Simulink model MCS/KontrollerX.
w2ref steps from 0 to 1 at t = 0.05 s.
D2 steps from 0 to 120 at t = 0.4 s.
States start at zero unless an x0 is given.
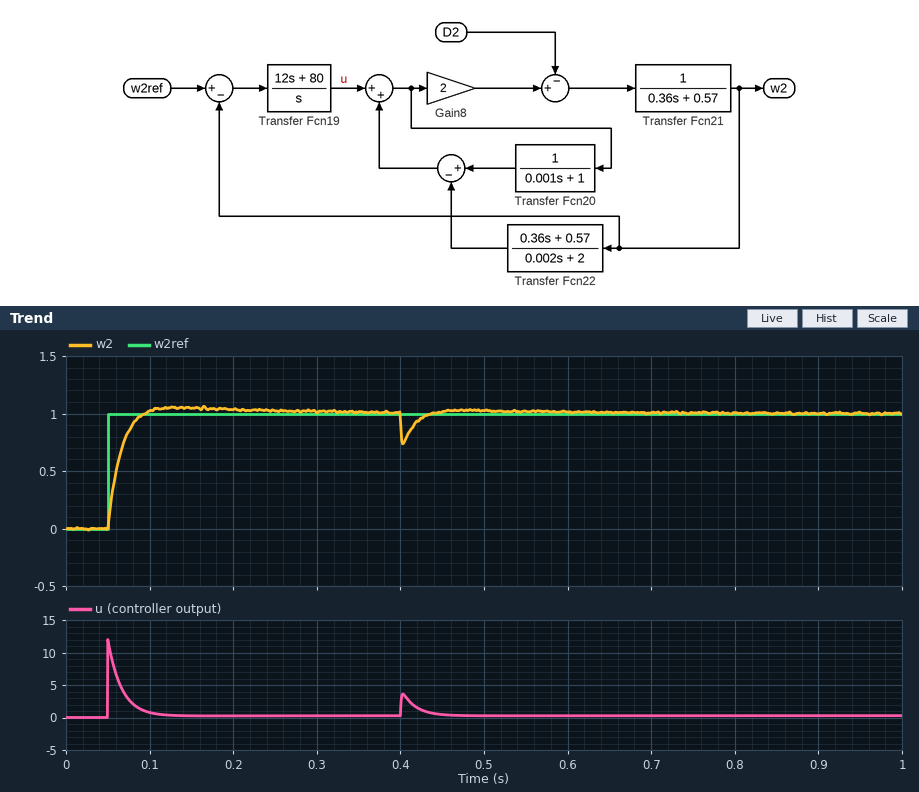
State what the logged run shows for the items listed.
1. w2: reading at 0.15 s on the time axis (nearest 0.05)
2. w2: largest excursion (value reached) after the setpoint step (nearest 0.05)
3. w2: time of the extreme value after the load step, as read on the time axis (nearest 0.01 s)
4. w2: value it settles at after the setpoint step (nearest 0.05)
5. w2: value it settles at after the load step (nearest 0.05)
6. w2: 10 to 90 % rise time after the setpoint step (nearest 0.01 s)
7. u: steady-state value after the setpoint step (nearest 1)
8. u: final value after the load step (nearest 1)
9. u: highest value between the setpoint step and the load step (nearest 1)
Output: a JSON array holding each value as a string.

["1.05", "1.05", "0.40 s", "1.00", "1.00", "0.03 s", "0", "0", "12"]
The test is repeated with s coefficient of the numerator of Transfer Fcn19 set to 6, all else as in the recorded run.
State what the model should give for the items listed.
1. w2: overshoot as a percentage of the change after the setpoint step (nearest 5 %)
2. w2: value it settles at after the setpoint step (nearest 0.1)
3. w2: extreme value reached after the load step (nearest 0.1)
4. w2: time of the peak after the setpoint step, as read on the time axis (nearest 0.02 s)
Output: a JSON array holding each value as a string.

["15 %", "1.0", "0.7", "0.16 s"]
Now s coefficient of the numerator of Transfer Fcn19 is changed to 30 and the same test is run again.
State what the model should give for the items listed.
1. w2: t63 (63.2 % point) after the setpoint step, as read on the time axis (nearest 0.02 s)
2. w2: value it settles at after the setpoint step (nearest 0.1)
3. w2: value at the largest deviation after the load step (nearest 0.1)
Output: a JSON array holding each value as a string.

["0.06 s", "1.0", "0.8"]
